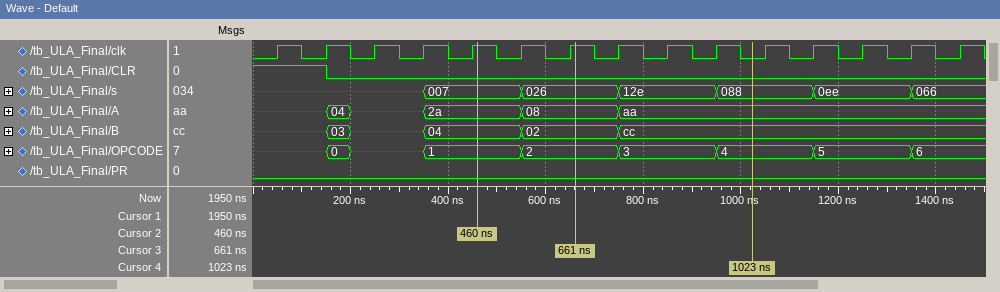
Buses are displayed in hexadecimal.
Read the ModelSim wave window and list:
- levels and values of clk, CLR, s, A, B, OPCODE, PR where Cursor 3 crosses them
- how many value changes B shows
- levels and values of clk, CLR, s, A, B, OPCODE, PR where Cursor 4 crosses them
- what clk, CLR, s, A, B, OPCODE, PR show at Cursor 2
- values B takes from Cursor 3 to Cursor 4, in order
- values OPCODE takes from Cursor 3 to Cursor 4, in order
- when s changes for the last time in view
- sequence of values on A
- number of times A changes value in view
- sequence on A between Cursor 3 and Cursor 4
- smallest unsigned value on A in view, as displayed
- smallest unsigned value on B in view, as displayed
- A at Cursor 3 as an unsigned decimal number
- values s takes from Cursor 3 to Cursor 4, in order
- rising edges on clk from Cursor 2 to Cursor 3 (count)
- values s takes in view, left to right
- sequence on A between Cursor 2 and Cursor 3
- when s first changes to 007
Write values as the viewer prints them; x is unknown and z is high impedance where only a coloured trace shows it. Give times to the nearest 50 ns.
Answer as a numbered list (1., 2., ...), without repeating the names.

1. clk=1, CLR=0, s=026, A=08, B=02, OPCODE=2, PR=0
2. 5
3. clk=0, CLR=0, s=088, A=aa, B=cc, OPCODE=4, PR=0
4. clk=1, CLR=0, s=007, A=2a, B=04, OPCODE=1, PR=0
5. 02, cc
6. 2, 3, 4
7. 1350 ns
8. x, 04, x, 2a, 08, aa
9. 5
10. 08, aa
11. 04
12. 02
13. 8
14. 026, 12e, 088
15. 2
16. x, 007, 026, 12e, 088, 0ee, 066
17. 2a, 08
18. 350 ns
